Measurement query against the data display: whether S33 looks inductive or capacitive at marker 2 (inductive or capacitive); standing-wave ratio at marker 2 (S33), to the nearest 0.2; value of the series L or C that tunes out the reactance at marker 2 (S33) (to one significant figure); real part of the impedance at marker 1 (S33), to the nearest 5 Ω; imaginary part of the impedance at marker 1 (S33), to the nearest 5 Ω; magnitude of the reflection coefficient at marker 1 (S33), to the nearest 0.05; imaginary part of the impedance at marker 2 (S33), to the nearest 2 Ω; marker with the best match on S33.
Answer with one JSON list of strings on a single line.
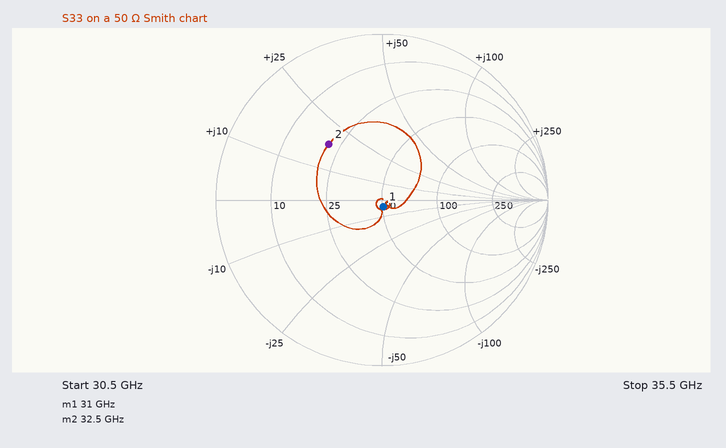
["inductive", "2.8", "300 fF", "50 Ω", "-5 Ω", "0.05", "+18 Ω", "marker 1"]
